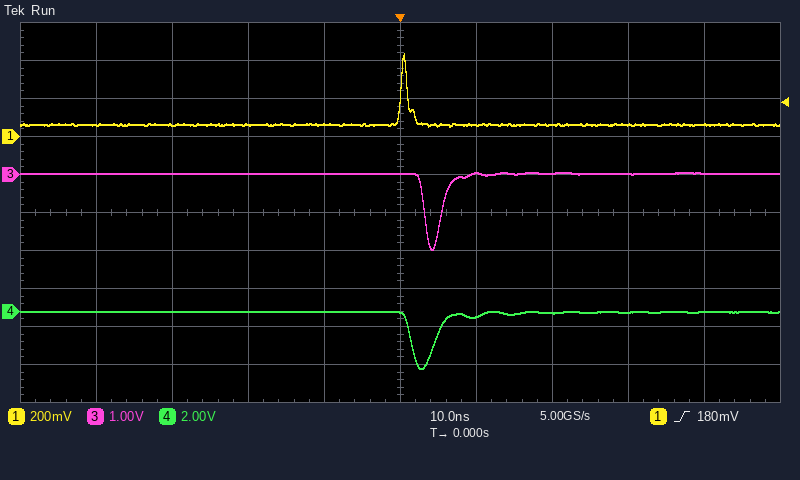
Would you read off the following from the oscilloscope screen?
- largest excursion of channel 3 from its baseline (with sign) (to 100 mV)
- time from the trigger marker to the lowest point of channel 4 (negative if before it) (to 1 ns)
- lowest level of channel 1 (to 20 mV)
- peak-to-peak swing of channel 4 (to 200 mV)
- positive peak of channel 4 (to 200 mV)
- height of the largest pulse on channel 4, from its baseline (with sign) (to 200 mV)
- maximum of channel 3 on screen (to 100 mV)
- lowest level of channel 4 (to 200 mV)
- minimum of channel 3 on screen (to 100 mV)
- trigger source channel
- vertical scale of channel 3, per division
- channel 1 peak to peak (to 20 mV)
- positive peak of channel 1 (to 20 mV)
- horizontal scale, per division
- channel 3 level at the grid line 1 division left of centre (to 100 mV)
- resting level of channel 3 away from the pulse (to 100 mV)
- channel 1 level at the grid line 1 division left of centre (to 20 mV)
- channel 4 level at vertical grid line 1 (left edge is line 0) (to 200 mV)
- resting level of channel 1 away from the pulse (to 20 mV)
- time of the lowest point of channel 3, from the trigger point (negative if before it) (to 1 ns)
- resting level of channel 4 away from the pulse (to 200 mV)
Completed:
-2.0 V
+3 ns
60 mV
3.0 V
0.0 V
-3.0 V
100 mV
-3.0 V
-2.0 V
channel 1
1 V
380 mV
440 mV
10 ns
0.0 V
0.0 V
60 mV
0.0 V
60 mV
+4 ns
0.0 V
